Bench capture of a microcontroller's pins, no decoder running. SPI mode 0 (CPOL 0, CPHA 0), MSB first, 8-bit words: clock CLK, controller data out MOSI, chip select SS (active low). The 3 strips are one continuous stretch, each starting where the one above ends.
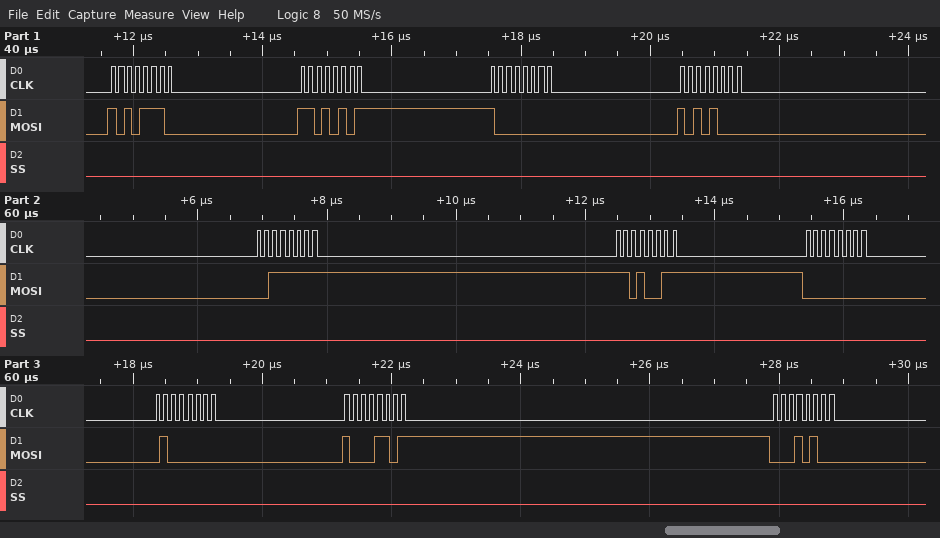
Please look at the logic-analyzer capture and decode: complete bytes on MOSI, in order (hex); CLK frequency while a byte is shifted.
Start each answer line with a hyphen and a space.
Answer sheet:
- AE D5 80 A8 3F D3 00 40 8D 14
- 8 MHz
